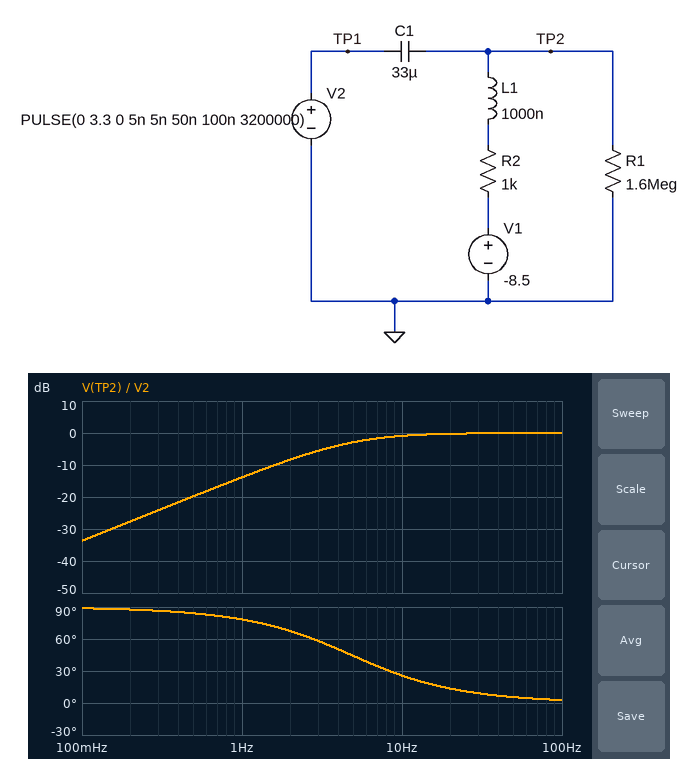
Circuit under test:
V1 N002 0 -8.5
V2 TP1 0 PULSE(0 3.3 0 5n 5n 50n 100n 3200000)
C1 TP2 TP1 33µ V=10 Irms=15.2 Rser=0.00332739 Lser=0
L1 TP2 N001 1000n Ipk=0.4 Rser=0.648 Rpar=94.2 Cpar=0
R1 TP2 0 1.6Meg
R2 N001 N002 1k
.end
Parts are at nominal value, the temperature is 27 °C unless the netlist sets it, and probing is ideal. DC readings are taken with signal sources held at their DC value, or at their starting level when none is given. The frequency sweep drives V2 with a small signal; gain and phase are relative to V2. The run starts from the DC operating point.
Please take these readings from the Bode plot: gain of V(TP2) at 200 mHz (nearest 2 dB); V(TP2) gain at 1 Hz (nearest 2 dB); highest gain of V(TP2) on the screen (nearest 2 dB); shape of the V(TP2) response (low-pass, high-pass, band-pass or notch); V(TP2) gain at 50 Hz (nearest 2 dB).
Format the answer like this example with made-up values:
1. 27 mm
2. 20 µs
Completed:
1. -28 dB
2. -14 dB
3. 0 dB
4. high-pass
5. 0 dB
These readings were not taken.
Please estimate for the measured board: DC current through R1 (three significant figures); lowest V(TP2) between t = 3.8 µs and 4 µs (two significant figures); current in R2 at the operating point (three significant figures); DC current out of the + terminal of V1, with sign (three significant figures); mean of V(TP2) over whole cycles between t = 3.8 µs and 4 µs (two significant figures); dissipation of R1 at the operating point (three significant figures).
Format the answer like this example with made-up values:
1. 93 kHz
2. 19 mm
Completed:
1. 5.31 µA
2. -8.5 V
3. 5.31 µA
4. -5.31 µA
5. -6.7 V
6. 45.1 µW
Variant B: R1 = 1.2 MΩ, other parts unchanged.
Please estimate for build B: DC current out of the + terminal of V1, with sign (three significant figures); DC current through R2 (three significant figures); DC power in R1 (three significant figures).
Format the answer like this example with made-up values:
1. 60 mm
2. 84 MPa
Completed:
1. -7.08 µA
2. 7.08 µA
3. 60.1 µW
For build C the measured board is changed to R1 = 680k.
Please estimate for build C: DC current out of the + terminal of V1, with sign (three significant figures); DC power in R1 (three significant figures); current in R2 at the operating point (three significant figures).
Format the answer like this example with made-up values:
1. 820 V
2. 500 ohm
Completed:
1. -12.5 µA
2. 106 µW
3. 12.5 µA
